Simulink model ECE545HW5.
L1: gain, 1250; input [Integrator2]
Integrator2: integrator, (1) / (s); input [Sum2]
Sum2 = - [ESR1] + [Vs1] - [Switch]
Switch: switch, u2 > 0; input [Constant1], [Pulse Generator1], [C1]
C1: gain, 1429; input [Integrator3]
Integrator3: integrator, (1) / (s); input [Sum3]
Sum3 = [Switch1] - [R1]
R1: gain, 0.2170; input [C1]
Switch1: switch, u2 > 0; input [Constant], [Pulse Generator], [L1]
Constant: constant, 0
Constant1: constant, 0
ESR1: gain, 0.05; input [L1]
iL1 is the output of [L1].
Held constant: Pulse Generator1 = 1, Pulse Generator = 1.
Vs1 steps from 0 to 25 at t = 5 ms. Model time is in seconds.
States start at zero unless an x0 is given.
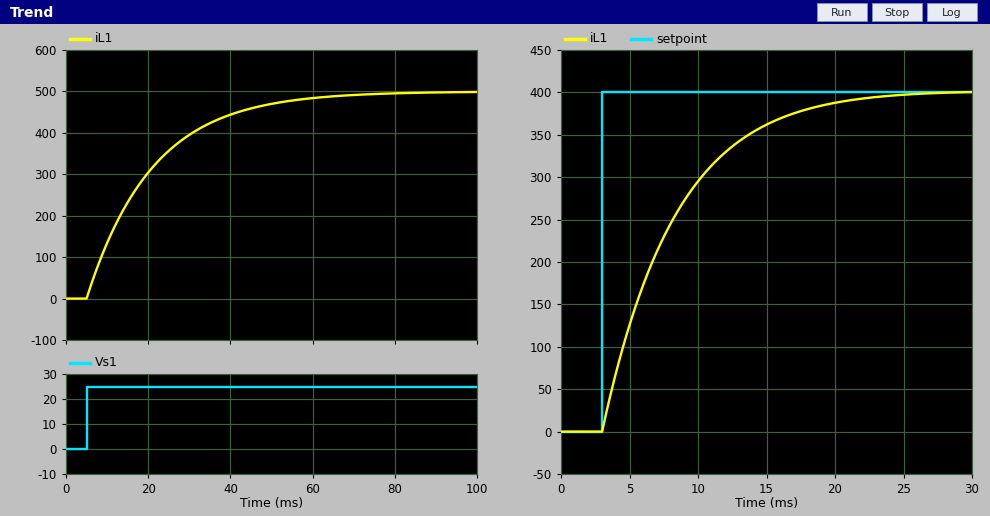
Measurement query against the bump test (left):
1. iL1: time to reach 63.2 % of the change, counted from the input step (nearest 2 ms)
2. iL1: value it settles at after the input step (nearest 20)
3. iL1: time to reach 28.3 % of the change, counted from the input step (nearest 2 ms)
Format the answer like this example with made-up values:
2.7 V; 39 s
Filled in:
16 ms; 500; 6 ms
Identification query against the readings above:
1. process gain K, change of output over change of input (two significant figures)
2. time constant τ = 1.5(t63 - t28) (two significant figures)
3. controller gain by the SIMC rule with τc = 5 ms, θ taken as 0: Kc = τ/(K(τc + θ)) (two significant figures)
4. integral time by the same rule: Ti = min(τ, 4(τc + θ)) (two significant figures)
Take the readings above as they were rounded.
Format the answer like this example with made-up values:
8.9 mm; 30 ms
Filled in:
20; 15 ms; 0.15; 15 ms
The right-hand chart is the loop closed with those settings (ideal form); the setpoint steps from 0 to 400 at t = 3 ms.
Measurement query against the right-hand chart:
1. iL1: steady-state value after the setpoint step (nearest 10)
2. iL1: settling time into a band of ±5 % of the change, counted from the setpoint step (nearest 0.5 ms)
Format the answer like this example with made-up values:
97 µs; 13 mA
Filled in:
400; 15.0 ms
